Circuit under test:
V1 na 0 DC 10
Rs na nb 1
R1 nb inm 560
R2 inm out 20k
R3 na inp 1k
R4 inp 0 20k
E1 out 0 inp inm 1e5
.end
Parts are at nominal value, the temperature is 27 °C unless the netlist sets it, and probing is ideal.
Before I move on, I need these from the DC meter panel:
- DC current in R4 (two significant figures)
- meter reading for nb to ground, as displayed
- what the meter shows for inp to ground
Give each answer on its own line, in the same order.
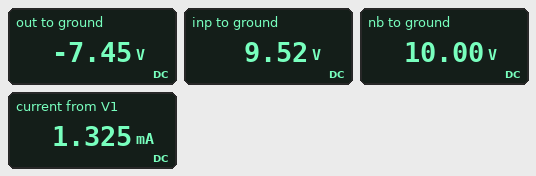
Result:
480 µA
10.00 V
9.52 V
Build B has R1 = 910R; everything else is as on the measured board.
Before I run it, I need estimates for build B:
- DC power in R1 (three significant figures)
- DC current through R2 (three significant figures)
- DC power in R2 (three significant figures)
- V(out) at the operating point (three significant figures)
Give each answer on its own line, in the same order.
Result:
249 µW
523 µA
5.46 mW
-930 mV
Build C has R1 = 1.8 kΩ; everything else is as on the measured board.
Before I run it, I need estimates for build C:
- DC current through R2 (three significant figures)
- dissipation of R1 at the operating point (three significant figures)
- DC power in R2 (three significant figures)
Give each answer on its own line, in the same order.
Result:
264 µA
126 µW
1.40 mW
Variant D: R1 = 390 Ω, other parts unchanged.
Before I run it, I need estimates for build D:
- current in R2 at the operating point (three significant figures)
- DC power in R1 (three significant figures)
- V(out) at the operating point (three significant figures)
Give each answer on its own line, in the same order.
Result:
1.22 mA
578 µW
-14.8 V
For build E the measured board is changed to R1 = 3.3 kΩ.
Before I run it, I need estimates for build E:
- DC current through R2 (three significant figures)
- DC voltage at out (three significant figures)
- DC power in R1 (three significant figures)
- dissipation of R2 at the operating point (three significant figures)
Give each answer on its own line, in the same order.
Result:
144 µA
6.64 V
68.7 µW
416 µW
